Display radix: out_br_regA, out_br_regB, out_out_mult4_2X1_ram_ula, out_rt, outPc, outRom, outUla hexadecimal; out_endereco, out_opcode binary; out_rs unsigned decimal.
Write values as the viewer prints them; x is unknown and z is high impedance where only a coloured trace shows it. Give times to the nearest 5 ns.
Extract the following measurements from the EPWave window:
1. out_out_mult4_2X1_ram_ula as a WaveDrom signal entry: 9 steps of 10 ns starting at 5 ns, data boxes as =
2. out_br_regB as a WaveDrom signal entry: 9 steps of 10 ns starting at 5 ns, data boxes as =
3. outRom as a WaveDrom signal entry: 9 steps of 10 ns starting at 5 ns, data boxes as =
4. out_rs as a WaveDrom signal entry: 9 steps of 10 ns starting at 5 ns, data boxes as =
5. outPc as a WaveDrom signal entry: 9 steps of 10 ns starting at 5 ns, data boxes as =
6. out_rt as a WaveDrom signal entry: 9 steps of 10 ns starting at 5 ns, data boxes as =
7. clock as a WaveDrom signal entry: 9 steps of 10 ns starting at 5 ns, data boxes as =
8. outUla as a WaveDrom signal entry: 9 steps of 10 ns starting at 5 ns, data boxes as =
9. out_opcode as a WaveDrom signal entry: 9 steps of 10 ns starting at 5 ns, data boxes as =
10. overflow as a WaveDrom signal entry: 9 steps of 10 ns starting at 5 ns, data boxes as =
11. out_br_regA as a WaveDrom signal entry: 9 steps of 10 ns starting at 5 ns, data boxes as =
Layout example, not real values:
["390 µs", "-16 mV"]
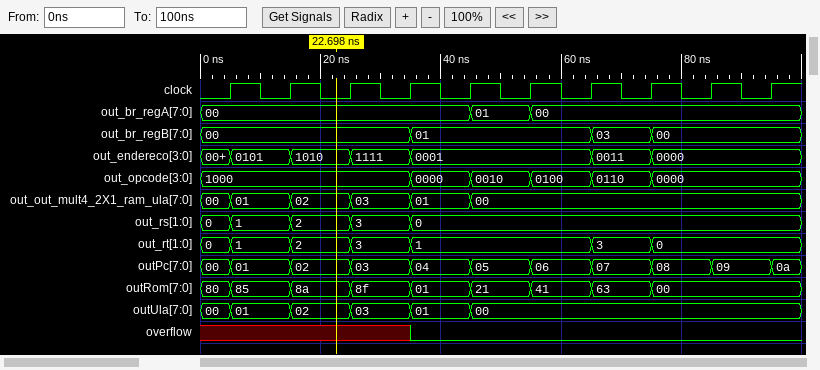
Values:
["{name: 'out_out_mult4_2X1_ram_ula', wave: '=====....', data: '01 02 03 01 00'}", "{name: 'out_br_regB', wave: '=..=..==.', data: '00 01 03 00'}", "{name: 'outRom', wave: '========.', data: '85 8a 8f 01 21 41 63 00'}", "{name: 'out_rs', wave: '====.....', data: '1 2 3 0'}", "{name: 'outPc', wave: '=========', data: '01 02 03 04 05 06 07 08 09'}", "{name: 'out_rt', wave: '====..==.', data: '1 2 3 1 3 0'}", "{name: 'clock', wave: 'p........'}", "{name: 'outUla', wave: '=====....', data: '01 02 03 01 00'}", "{name: 'out_opcode', wave: '=..=====.', data: '1000 0000 0010 0100 0110 0000'}", "{name: 'overflow', wave: 'x..0.....'}", "{name: 'out_br_regA', wave: '=...==...', data: '00 01 00'}"]
